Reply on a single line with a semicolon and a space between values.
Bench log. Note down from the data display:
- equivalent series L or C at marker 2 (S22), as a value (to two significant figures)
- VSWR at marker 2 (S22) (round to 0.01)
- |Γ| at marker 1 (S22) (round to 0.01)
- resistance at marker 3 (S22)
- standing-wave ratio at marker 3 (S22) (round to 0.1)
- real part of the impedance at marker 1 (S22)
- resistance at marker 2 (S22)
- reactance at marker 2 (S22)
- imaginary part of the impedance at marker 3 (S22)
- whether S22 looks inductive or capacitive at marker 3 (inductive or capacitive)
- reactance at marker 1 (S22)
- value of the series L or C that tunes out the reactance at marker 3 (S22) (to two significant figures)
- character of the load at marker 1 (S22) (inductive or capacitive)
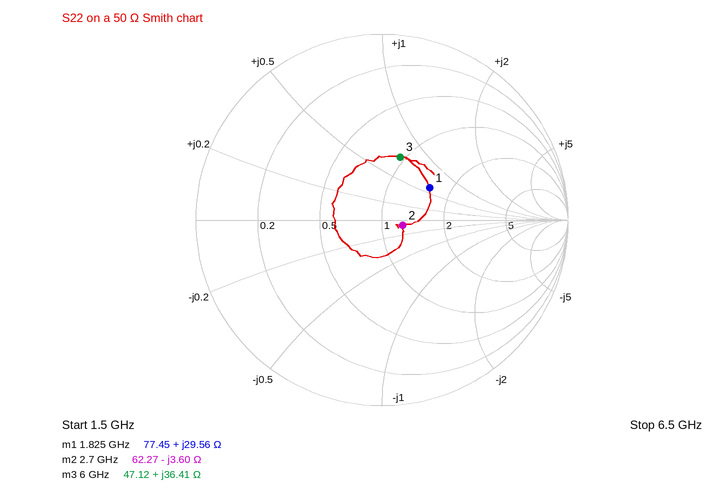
16 pF; 1.26; 0.31; 47.12 Ω; 2.1; 77.45 Ω; 62.27 Ω; -3.60 Ω; +36.41 Ω; inductive; +29.56 Ω; 730 fF; inductive
